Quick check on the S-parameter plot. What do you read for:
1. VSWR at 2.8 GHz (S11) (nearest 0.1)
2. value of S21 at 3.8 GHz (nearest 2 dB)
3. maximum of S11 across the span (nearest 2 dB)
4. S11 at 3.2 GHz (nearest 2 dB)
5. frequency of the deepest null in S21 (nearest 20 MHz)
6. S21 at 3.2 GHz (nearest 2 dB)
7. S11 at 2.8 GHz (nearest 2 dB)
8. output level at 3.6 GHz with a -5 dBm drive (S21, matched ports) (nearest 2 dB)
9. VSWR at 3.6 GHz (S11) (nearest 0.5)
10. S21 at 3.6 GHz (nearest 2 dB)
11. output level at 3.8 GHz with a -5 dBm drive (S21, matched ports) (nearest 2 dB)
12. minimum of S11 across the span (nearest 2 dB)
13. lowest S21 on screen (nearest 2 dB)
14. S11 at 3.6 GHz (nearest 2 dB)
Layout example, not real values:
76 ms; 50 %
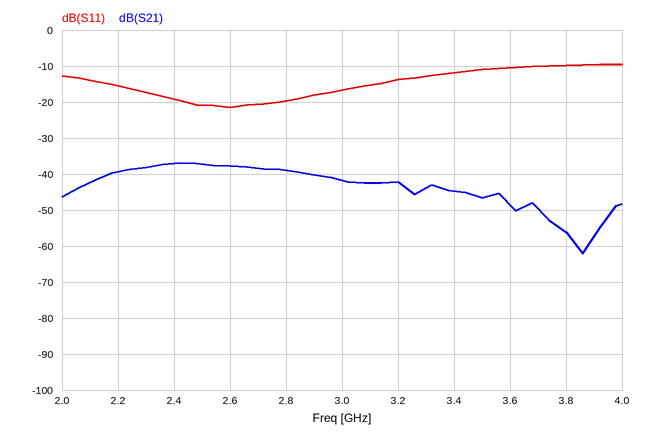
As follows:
1.2; -56 dB; -10 dB; -14 dB; 3.86 GHz; -42 dB; -20 dB; -54 dBm; 2.0; -48 dB; -62 dBm; -22 dB; -62 dB; -10 dB
